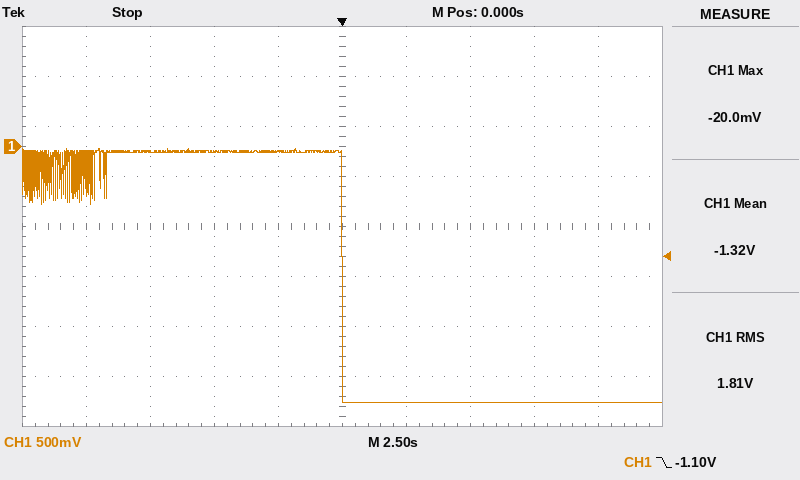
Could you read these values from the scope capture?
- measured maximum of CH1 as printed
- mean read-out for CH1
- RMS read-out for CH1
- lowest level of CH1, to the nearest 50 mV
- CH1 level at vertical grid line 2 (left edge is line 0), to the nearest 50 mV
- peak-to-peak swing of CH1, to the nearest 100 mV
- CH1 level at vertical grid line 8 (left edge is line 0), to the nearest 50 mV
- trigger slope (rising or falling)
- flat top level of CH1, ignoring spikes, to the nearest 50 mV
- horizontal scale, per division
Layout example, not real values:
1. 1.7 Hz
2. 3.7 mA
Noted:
1. -20.0 mV
2. -1.32 V
3. 1.81 V
4. -2.55 V
5. -50 mV
6. 2.50 V
7. -2.55 V
8. falling
9. -50 mV
10. 2.5 s
